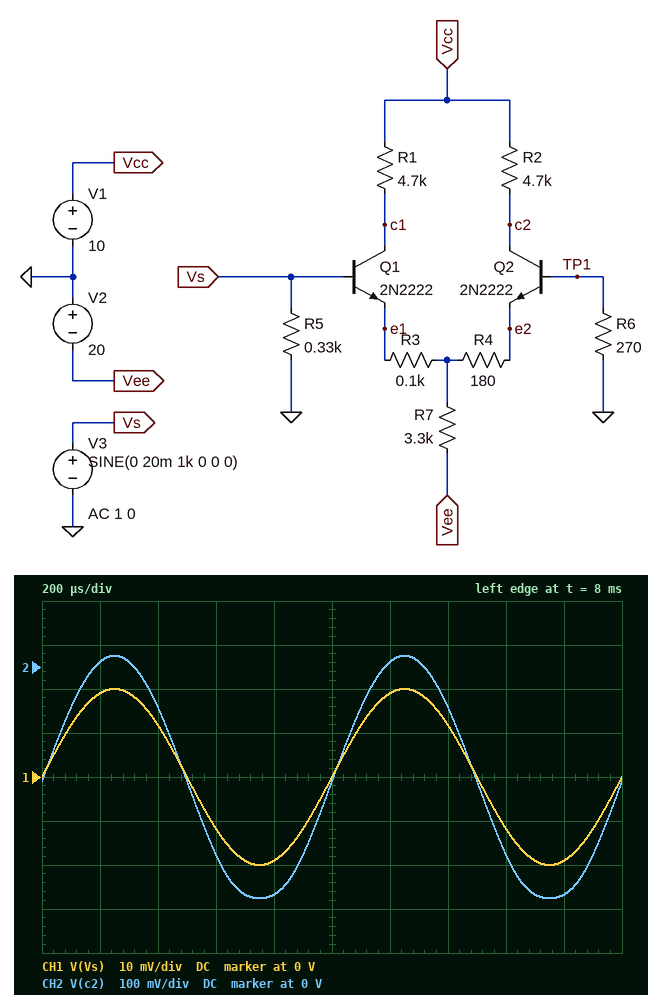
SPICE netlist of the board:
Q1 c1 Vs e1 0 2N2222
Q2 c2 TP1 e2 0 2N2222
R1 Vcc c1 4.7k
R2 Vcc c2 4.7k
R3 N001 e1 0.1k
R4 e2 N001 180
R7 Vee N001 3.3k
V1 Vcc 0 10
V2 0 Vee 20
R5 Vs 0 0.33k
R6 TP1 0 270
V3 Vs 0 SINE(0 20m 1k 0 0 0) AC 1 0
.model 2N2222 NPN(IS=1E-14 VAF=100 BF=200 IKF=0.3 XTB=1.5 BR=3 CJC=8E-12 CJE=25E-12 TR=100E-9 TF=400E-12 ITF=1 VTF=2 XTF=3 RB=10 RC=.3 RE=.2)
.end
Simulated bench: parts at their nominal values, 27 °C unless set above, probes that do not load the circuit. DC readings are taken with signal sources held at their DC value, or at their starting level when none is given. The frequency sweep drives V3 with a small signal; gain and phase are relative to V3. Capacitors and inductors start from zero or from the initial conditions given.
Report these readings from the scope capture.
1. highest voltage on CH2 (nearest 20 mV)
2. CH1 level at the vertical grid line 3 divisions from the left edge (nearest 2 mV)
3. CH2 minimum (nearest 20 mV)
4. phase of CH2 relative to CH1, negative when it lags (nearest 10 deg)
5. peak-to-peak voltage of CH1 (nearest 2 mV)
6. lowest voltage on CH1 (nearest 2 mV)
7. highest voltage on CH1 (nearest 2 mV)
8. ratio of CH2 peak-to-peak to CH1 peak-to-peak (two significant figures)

20 mV
-12 mV
-520 mV
0 deg
40 mV
-20 mV
20 mV
14
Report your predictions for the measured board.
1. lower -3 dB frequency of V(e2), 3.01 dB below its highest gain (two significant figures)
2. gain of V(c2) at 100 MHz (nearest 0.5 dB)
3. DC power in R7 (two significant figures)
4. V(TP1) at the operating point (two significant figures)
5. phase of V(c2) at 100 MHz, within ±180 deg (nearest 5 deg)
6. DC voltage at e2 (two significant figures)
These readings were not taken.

1.8 MHz
-8.0 dB
110 mW
-3.0 mV
-30 deg
-680 mV
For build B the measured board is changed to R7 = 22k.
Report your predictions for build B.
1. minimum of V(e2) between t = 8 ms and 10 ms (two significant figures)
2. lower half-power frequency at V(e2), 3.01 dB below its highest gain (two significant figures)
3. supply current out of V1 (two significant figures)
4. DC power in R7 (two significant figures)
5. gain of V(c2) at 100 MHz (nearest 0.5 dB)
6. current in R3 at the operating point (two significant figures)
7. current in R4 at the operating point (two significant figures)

-630 mV
4.0 MHz
870 µA
17 mW
-13.5 dB
530 µA
350 µA
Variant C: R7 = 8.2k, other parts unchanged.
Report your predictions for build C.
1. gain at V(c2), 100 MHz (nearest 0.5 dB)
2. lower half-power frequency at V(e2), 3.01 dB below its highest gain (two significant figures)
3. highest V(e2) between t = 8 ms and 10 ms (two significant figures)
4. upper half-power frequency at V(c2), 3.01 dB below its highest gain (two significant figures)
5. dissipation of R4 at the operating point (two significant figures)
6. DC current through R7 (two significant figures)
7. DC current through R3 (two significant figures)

-9.0 dB
4.1 MHz
-650 mV
4.3 MHz
140 µW
2.3 mA
1.5 mA
